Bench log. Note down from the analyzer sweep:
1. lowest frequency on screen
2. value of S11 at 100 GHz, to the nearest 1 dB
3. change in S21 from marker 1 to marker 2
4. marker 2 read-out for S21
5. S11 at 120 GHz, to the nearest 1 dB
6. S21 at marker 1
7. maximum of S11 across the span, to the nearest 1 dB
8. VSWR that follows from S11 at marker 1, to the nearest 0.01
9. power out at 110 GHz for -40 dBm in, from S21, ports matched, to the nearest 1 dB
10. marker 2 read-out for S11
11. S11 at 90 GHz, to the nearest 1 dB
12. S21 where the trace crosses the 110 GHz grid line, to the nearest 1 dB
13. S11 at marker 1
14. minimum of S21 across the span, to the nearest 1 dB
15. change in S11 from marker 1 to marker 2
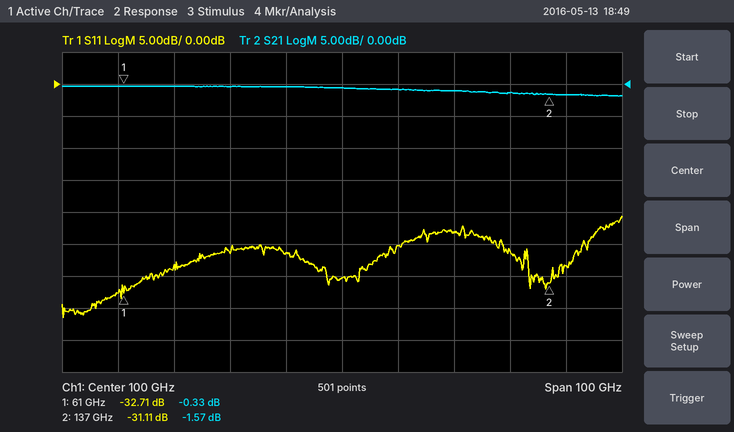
50 GHz
-30 dB
-1.24 dB
-1.57 dB
-23 dB
-0.33 dB
-21 dB
1.05
-41 dBm
-31.11 dB
-26 dB
-1 dB
-32.71 dB
-2 dB
1.60 dB
